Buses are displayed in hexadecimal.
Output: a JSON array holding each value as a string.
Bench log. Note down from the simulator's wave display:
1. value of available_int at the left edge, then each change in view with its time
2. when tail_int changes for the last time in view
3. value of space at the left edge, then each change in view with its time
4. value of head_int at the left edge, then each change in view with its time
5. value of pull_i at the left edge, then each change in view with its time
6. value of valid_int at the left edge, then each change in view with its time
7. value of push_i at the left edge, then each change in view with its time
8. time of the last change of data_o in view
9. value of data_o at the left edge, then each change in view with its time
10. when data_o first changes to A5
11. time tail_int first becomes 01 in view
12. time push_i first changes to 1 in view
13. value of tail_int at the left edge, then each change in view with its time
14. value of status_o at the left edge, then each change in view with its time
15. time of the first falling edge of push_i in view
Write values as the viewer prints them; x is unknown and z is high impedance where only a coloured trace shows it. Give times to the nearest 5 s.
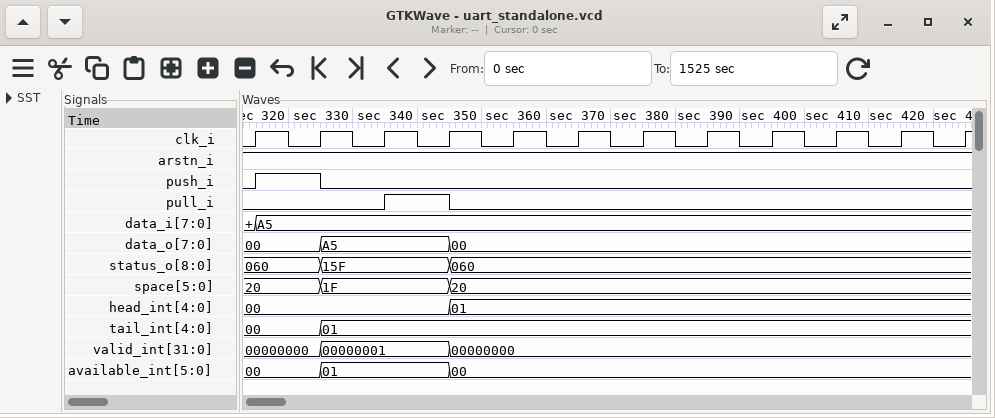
["00, 01 at 325 s, 00 at 345 s", "325 s", "20, 1F at 325 s, 20 at 345 s", "00, 01 at 345 s", "0, 1 at 335 s, 0 at 345 s", "00000000, 00000001 at 325 s, 00000000 at 345 s", "0, 1 at 315 s, 0 at 325 s", "345 s", "00, A5 at 325 s, 00 at 345 s", "325 s", "325 s", "315 s", "00, 01 at 325 s", "060, 15F at 325 s, 060 at 345 s", "325 s"]
